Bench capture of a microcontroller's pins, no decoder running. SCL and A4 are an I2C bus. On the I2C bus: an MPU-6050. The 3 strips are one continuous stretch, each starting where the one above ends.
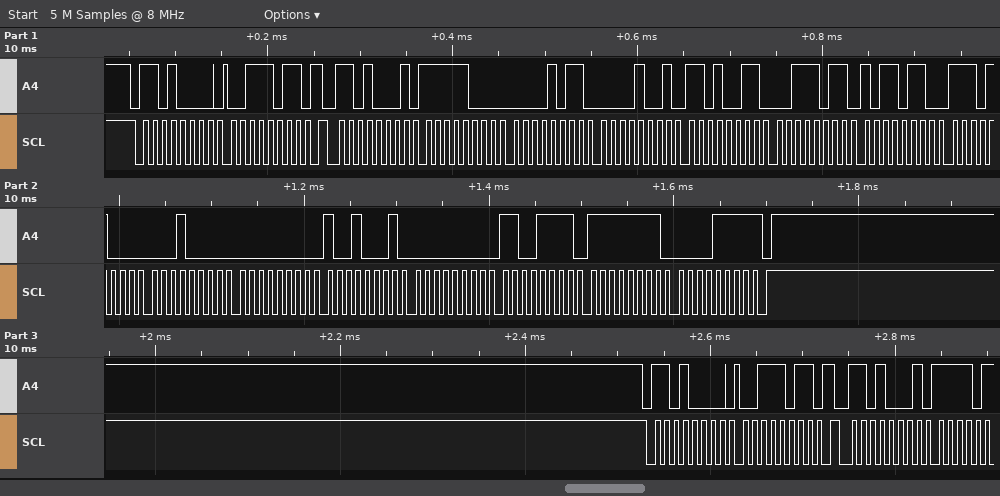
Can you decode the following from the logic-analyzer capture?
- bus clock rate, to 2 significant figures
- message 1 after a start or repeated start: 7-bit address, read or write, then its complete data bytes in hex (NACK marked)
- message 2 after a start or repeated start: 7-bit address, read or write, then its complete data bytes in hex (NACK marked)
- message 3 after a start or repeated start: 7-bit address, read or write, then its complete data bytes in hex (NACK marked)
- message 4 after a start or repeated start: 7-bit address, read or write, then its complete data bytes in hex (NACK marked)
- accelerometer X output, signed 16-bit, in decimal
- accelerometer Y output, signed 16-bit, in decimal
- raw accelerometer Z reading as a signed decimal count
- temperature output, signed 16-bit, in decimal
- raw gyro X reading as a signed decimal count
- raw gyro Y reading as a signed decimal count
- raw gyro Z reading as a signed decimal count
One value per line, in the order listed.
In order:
100 kHz
0x68 write: 3B
0x68 read: F8 0B 09 D3 3B B6 E8 10 00 91 00 CF FF 0F NACK
0x68 write: 3B
0x68 read
-2037
2515
15286
-6128
145
207
-241
